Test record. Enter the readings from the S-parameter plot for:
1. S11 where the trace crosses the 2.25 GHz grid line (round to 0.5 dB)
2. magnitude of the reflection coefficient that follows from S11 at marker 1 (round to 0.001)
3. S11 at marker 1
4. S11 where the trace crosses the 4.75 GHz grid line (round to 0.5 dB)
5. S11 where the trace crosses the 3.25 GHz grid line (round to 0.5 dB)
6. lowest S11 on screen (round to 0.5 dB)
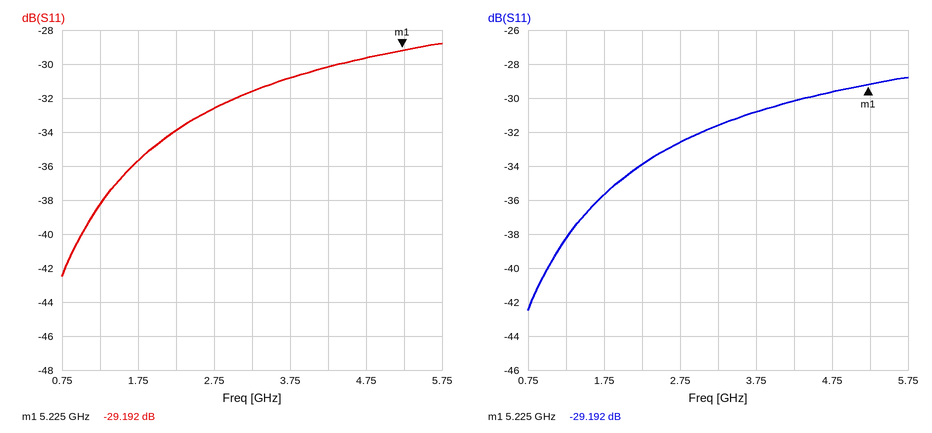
-34.0 dB
0.035
-29.192 dB
-29.5 dB
-31.5 dB
-42.5 dB
